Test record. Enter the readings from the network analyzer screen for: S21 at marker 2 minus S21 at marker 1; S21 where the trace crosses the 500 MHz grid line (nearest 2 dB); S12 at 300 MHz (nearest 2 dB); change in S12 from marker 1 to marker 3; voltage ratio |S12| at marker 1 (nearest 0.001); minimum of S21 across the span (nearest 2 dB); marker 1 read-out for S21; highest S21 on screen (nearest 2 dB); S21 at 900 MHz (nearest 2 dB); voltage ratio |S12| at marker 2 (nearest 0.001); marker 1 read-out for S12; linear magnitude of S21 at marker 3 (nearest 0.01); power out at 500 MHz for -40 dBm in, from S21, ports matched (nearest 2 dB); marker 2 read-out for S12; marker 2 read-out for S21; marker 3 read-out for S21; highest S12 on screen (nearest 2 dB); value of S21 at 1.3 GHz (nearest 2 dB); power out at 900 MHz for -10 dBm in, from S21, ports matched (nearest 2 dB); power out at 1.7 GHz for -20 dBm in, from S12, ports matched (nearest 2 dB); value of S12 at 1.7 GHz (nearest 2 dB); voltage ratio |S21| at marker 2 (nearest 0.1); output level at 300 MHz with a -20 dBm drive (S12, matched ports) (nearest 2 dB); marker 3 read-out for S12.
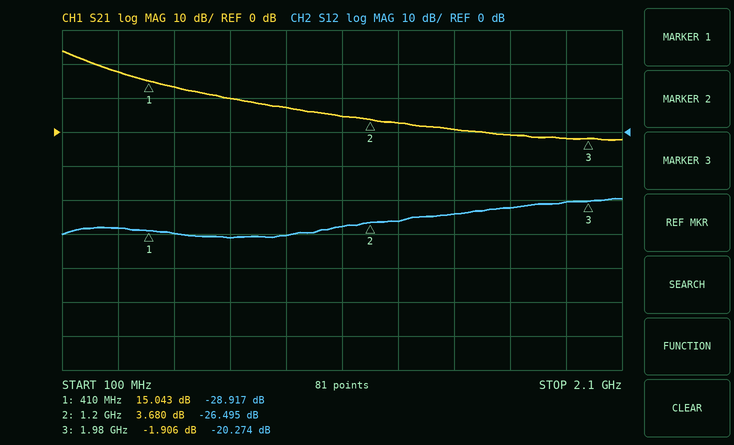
-11.363 dB
14 dB
-28 dB
8.643 dB
0.036
-2 dB
15.043 dB
24 dB
8 dB
0.047
-28.917 dB
0.80
-26 dBm
-26.495 dB
3.680 dB
-1.906 dB
-20 dB
2 dB
-2 dBm
-42 dBm
-22 dB
1.5
-48 dBm
-20.274 dB
